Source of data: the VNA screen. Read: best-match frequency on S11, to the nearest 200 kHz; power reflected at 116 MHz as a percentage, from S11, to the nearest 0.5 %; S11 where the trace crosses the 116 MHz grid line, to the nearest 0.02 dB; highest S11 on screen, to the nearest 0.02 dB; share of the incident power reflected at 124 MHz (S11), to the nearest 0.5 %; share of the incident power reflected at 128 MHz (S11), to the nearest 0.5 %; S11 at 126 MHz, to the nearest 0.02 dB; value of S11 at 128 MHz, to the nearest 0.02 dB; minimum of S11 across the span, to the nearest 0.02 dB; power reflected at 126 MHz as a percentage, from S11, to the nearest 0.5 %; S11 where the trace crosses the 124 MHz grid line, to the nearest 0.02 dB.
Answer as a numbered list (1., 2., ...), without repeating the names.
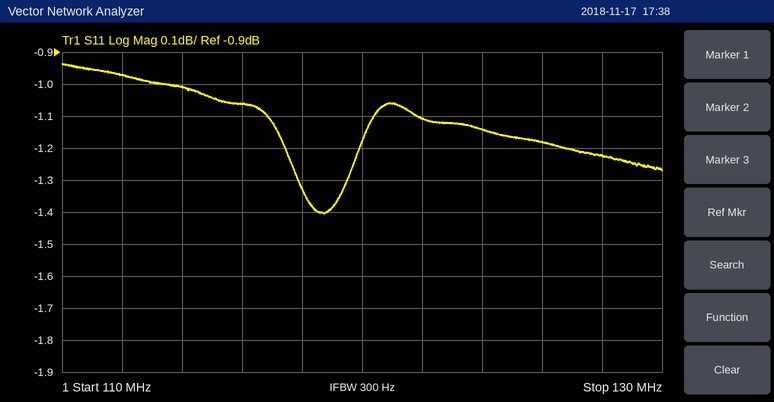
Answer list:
1. 118.8 MHz
2. 78.5 %
3. -1.06 dB
4. -0.94 dB
5. 77.0 %
6. 75.5 %
7. -1.18 dB
8. -1.22 dB
9. -1.40 dB
10. 76.0 %
11. -1.14 dB
